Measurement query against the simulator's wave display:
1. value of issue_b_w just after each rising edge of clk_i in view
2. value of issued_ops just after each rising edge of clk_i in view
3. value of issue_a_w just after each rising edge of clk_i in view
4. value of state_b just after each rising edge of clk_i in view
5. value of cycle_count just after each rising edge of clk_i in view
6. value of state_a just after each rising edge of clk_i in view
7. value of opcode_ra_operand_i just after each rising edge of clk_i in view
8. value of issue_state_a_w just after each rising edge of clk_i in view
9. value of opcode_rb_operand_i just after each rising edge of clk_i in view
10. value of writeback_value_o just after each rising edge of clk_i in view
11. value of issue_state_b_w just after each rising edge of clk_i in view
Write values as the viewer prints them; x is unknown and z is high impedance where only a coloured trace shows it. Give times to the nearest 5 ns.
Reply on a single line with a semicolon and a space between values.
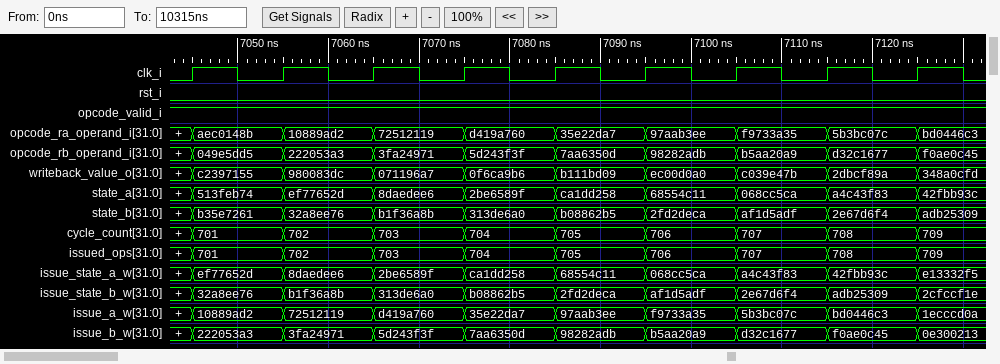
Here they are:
222053a3, 3fa24971, 5d243f3f, 7aa6350d, 98282adb, b5aa20a9, d32c1677, f0ae0c45, 0e300213; 701, 702, 703, 704, 705, 706, 707, 708, 709; 10889ad2, 72512119, d419a760, 35e22da7, 97aab3ee, f9733a35, 5b3bc07c, bd0446c3, 1ecccd0a; b35e7261, 32a8ee76, b1f36a8b, 313de6a0, b08862b5, 2fd2deca, af1d5adf, 2e67d6f4, adb25309; 701, 702, 703, 704, 705, 706, 707, 708, 709; 513feb74, ef77652d, 8daedee6, 2be6589f, ca1dd258, 68554c11, 068cc5ca, a4c43f83, 42fbb93c; aec0148b, 10889ad2, 72512119, d419a760, 35e22da7, 97aab3ee, f9733a35, 5b3bc07c, bd0446c3; ef77652d, 8daedee6, 2be6589f, ca1dd258, 68554c11, 068cc5ca, a4c43f83, 42fbb93c, e13332f5; 049e5dd5, 222053a3, 3fa24971, 5d243f3f, 7aa6350d, 98282adb, b5aa20a9, d32c1677, f0ae0c45; c2397155, 980083dc, 071196a7, 0f6ca9b6, b111bd09, ec00d0a0, c039e47b, 2dbcf89a, 348a0cfd; 32a8ee76, b1f36a8b, 313de6a0, b08862b5, 2fd2deca, af1d5adf, 2e67d6f4, adb25309, 2cfccf1e
